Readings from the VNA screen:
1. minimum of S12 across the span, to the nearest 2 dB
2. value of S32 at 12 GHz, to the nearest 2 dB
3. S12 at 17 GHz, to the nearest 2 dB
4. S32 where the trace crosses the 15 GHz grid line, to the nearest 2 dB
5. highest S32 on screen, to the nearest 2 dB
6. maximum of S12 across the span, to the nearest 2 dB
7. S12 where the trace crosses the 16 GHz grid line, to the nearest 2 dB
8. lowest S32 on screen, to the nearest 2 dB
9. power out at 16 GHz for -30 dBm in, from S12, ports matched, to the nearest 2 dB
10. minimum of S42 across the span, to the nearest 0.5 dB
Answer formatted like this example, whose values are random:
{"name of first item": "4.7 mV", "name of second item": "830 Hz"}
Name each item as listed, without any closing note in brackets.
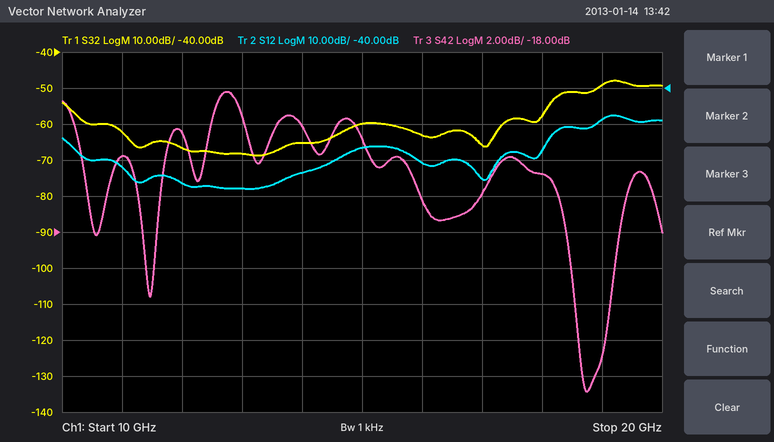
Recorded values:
{"minimum of S12 across the span, to the nearest 2 dB": "-68 dB", "value of S32 at 12 GHz, to the nearest 2 dB": "-66 dB", "S12 at 17 GHz, to the nearest 2 dB": "-66 dB", "S32 where the trace crosses the 15 GHz grid line, to the nearest 2 dB": "-60 dB", "highest S32 on screen, to the nearest 2 dB": "-48 dB", "maximum of S12 across the span, to the nearest 2 dB": "-48 dB", "S12 where the trace crosses the 16 GHz grid line, to the nearest 2 dB": "-60 dB", "lowest S32 on screen, to the nearest 2 dB": "-68 dB", "power out at 16 GHz for -30 dBm in, from S12, ports matched, to the nearest 2 dB": "-90 dBm", "minimum of S42 across the span, to the nearest 0.5 dB": "-27.0 dB"}
